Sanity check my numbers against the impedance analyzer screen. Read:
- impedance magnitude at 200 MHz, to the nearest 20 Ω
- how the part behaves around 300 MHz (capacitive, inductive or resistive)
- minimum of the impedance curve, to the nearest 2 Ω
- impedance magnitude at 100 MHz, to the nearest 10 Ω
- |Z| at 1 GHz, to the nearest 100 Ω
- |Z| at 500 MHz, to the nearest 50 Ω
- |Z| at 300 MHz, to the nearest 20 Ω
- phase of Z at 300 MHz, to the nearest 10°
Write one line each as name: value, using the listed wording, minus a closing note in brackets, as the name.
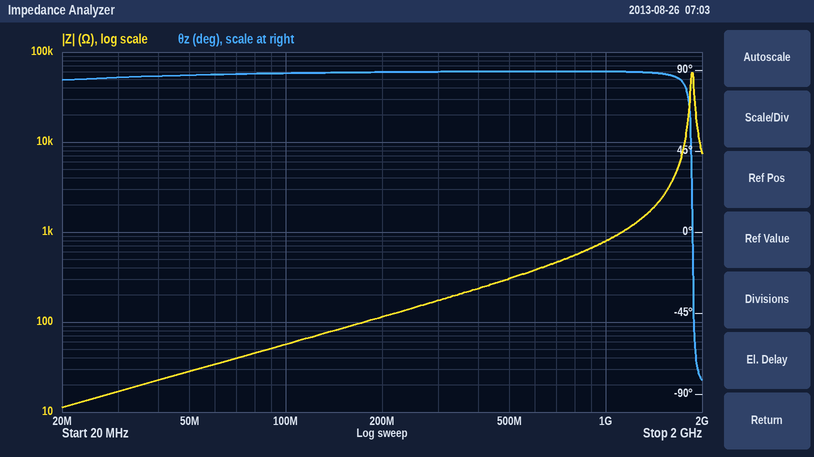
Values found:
impedance magnitude at 200 MHz, to the nearest 20 Ω: 120 Ω
how the part behaves around 300 MHz: inductive
minimum of the impedance curve, to the nearest 2 Ω: 12 Ω
impedance magnitude at 100 MHz, to the nearest 10 Ω: 60 Ω
|Z| at 1 GHz, to the nearest 100 Ω: 800 Ω
|Z| at 500 MHz, to the nearest 50 Ω: 300 Ω
|Z| at 300 MHz, to the nearest 20 Ω: 180 Ω
phase of Z at 300 MHz, to the nearest 10°: 90°
